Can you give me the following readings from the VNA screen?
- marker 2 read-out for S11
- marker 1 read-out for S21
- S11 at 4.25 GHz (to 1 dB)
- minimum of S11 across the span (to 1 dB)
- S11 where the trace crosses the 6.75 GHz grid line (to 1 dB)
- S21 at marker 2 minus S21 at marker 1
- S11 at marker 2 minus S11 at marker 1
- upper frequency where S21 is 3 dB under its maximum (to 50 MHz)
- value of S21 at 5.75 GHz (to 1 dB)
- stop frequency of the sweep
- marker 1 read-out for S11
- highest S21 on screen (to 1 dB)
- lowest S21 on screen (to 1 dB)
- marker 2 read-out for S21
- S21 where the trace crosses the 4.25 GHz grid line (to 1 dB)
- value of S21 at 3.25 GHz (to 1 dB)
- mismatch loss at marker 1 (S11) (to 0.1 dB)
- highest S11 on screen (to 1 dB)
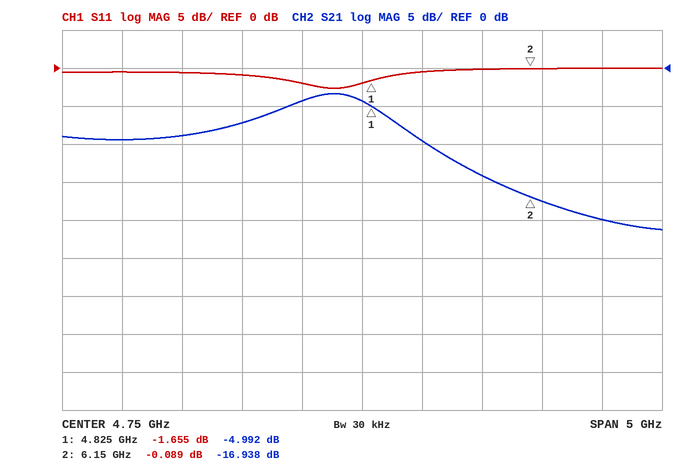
-0.089 dB
-4.992 dB
-2 dB
-3 dB
0 dB
-11.946 dB
1.566 dB
4.95 GHz
-14 dB
7.25 GHz
-1.655 dB
-3 dB
-21 dB
-16.938 dB
-4 dB
-9 dB
5.0 dB
0 dB
